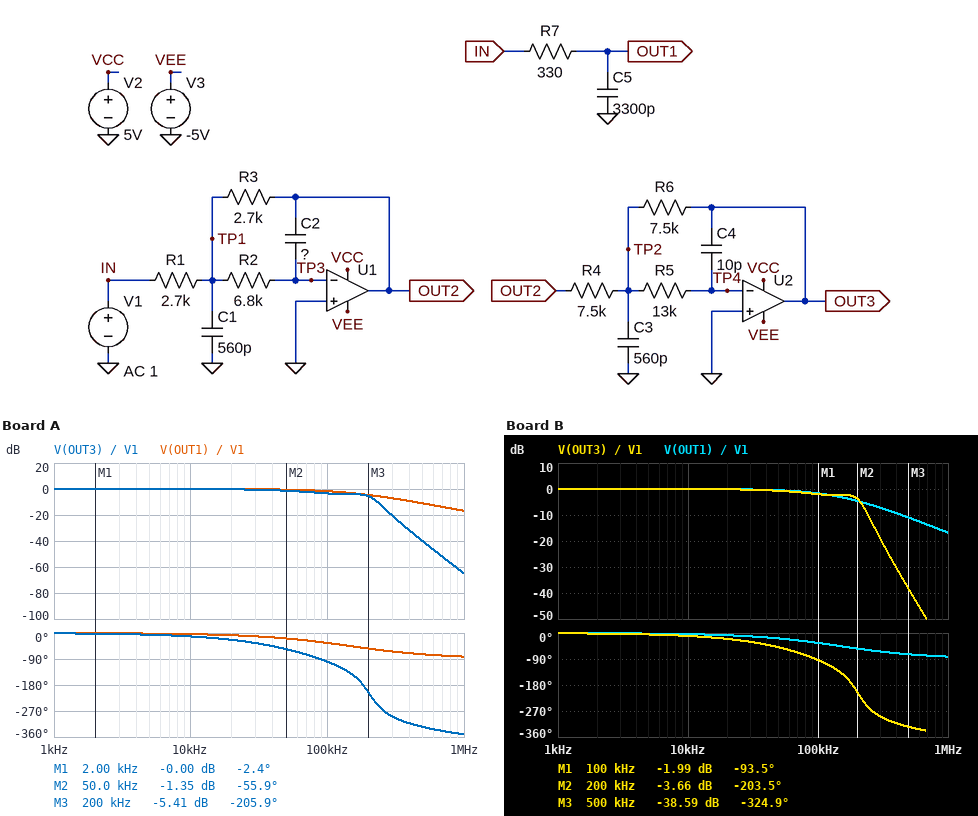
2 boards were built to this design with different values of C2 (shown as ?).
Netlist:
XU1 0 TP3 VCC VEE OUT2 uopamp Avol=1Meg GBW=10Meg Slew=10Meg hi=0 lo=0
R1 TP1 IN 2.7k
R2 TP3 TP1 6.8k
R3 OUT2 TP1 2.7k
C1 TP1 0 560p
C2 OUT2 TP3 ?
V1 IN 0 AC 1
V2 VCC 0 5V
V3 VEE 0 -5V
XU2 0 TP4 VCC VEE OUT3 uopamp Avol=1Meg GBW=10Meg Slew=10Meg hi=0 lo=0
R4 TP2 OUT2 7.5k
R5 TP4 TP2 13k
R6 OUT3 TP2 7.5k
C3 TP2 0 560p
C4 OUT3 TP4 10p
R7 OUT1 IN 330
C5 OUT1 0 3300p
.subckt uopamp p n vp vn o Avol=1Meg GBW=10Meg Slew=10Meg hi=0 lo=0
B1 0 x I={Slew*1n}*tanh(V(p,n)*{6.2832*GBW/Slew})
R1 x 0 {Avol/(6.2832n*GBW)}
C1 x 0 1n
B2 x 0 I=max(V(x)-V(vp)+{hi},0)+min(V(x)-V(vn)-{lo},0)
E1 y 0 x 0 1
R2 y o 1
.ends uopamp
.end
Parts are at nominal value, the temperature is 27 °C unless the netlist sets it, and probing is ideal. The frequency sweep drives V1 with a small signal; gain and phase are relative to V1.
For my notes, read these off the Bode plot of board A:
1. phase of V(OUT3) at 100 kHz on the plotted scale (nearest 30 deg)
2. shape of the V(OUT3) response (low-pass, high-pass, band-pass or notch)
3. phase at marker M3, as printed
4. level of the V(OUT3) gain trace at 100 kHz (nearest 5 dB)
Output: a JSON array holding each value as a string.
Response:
["-90 deg", "low-pass", "-205.9 deg", "-5 dB"]
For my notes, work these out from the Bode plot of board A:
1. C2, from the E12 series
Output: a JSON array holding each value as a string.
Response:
["180 pF"]
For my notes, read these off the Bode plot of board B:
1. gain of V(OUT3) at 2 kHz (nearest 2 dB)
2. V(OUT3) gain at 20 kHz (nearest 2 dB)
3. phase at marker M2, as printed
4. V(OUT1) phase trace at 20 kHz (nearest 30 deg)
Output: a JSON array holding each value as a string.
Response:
["0 dB", "0 dB", "-203.5 deg", "0 deg"]
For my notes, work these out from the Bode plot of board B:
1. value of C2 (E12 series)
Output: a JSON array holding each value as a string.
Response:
["150 pF"]
